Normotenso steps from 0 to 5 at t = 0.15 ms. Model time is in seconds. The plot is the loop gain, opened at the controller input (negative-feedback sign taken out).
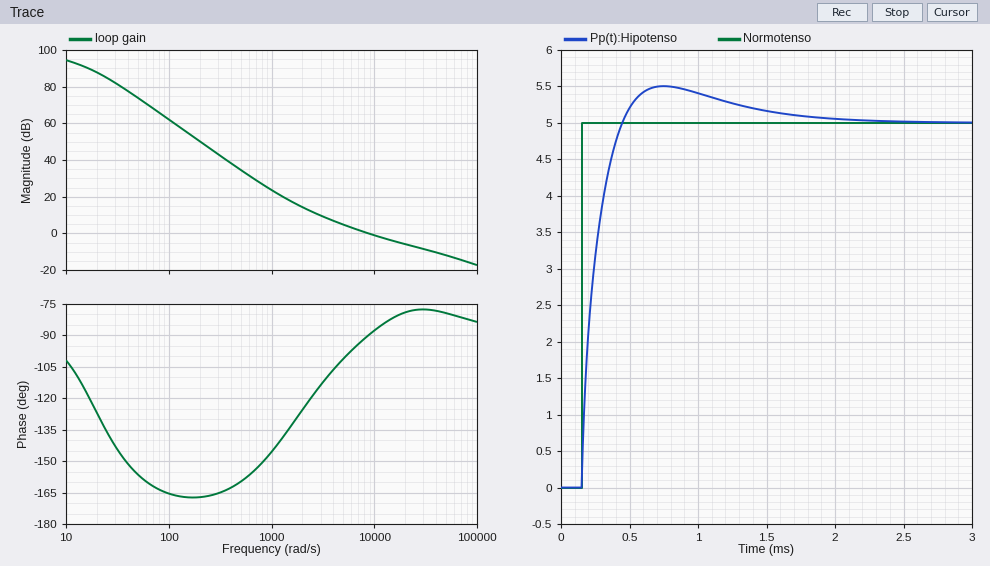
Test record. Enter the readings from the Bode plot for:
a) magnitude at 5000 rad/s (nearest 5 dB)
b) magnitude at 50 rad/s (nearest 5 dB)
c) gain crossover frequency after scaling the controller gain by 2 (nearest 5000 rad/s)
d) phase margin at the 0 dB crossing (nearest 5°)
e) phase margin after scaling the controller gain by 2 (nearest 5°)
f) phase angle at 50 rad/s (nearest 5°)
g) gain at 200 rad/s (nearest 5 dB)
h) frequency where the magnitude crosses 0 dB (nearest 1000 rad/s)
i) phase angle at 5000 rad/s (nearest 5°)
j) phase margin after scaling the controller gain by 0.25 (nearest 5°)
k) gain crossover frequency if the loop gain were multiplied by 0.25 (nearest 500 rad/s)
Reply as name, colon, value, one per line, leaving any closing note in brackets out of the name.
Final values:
magnitude at 5000 rad/s: 5 dB
magnitude at 50 rad/s: 75 dB
gain crossover frequency after scaling the controller gain by 2: 20000 rad/s
phase margin at the 0 dB crossing: 90°
phase margin after scaling the controller gain by 2: 100°
phase angle at 50 rad/s: -155°
gain at 200 rad/s: 50 dB
frequency where the magnitude crosses 0 dB: 9000 rad/s
phase angle at 5000 rad/s: -100°
phase margin after scaling the controller gain by 0.25: 60°
gain crossover frequency if the loop gain were multiplied by 0.25: 2500 rad/s
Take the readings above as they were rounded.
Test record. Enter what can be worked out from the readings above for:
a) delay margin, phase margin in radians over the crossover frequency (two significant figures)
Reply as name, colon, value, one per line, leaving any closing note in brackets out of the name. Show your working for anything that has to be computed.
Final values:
delay margin, phase margin in radians over the crossover frequency: 90 × π / 180 / 9000 = 0.00017 s
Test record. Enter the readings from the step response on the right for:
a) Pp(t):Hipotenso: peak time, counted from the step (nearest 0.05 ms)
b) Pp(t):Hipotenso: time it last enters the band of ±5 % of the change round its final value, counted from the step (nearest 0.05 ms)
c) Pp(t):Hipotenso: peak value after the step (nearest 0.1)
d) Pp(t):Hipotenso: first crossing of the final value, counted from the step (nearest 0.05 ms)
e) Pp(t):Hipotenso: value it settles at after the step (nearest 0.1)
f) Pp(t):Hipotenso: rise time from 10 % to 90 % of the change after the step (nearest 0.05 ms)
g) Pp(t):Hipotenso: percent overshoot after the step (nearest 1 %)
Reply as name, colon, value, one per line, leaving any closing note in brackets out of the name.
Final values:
Pp(t):Hipotenso: peak time, counted from the step: 0.60 ms
Pp(t):Hipotenso: time it last enters the band of ±5 % of the change round its final value, counted from the step: 1.15 ms
Pp(t):Hipotenso: peak value after the step: 5.5
Pp(t):Hipotenso: first crossing of the final value, counted from the step: 0.30 ms
Pp(t):Hipotenso: value it settles at after the step: 5.0
Pp(t):Hipotenso: rise time from 10 % to 90 % of the change after the step: 0.20 ms
Pp(t):Hipotenso: percent overshoot after the step: 10 %
